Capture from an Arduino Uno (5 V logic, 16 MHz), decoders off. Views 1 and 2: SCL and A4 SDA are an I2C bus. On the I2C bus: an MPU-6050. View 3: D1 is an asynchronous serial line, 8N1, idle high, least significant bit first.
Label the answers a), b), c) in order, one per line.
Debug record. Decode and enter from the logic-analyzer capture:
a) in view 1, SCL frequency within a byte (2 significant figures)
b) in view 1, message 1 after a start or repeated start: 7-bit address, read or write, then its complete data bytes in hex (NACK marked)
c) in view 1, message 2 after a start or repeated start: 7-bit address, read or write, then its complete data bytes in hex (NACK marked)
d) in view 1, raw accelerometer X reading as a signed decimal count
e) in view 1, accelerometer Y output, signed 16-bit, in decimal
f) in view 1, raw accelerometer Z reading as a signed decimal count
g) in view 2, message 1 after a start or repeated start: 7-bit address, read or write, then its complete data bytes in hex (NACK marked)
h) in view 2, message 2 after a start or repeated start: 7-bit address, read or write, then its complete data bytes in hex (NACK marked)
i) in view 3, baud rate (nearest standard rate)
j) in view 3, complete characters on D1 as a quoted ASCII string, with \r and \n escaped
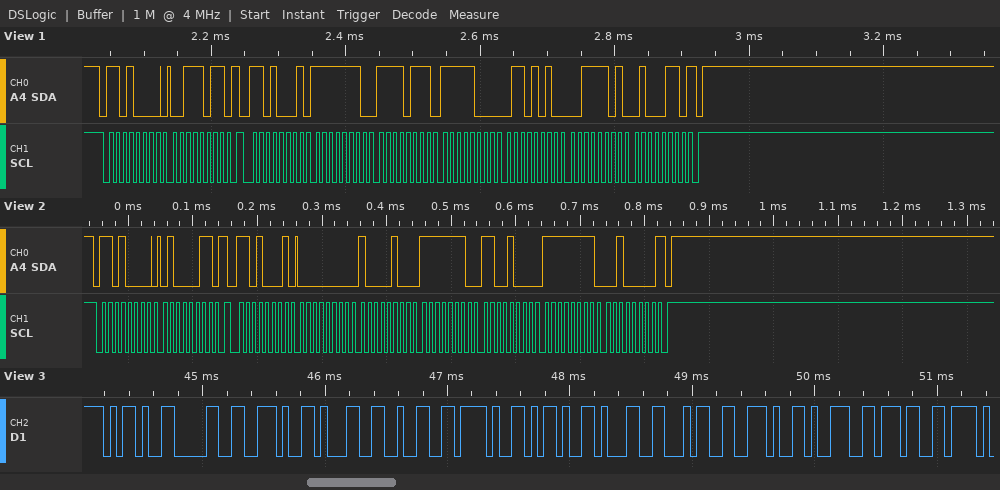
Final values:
a) 100 kHz
b) 0x68 write: 3B
c) 0x68 read: FE F7 F8 6A 3D 46 NACK
d) -265
e) -1942
f) 15686
g) 0x68 write: 43
h) 0x68 read: 00 84 FE C8 FF 20 NACK
i) 19200 baud
j) "-0.12/-14.97"
